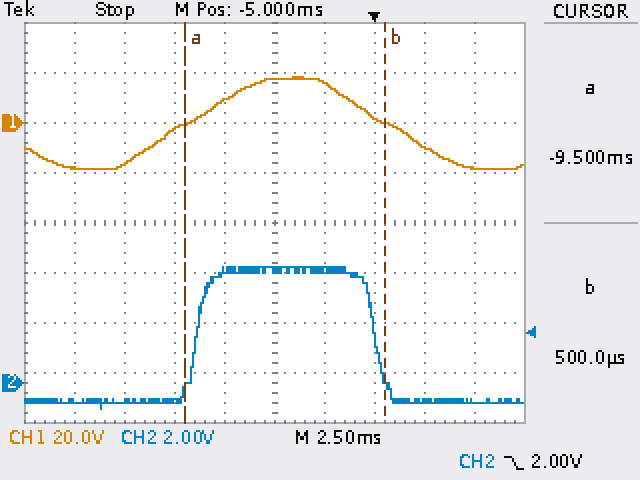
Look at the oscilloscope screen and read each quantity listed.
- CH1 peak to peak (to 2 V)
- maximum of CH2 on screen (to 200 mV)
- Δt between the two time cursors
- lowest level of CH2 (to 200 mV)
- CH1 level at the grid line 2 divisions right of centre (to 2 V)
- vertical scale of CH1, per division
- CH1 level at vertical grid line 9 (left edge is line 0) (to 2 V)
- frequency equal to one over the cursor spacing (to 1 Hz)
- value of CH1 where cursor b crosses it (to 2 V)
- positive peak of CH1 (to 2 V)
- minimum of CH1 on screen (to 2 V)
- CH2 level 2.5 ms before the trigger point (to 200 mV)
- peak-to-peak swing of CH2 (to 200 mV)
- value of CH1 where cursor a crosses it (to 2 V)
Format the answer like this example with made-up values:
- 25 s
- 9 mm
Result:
- 36 V
- 4.6 V
- 10.00 ms
- -1.0 V
- 2 V
- 20 V
- -18 V
- 100 Hz
- 0 V
- 18 V
- -18 V
- 4.6 V
- 5.6 V
- 0 V
